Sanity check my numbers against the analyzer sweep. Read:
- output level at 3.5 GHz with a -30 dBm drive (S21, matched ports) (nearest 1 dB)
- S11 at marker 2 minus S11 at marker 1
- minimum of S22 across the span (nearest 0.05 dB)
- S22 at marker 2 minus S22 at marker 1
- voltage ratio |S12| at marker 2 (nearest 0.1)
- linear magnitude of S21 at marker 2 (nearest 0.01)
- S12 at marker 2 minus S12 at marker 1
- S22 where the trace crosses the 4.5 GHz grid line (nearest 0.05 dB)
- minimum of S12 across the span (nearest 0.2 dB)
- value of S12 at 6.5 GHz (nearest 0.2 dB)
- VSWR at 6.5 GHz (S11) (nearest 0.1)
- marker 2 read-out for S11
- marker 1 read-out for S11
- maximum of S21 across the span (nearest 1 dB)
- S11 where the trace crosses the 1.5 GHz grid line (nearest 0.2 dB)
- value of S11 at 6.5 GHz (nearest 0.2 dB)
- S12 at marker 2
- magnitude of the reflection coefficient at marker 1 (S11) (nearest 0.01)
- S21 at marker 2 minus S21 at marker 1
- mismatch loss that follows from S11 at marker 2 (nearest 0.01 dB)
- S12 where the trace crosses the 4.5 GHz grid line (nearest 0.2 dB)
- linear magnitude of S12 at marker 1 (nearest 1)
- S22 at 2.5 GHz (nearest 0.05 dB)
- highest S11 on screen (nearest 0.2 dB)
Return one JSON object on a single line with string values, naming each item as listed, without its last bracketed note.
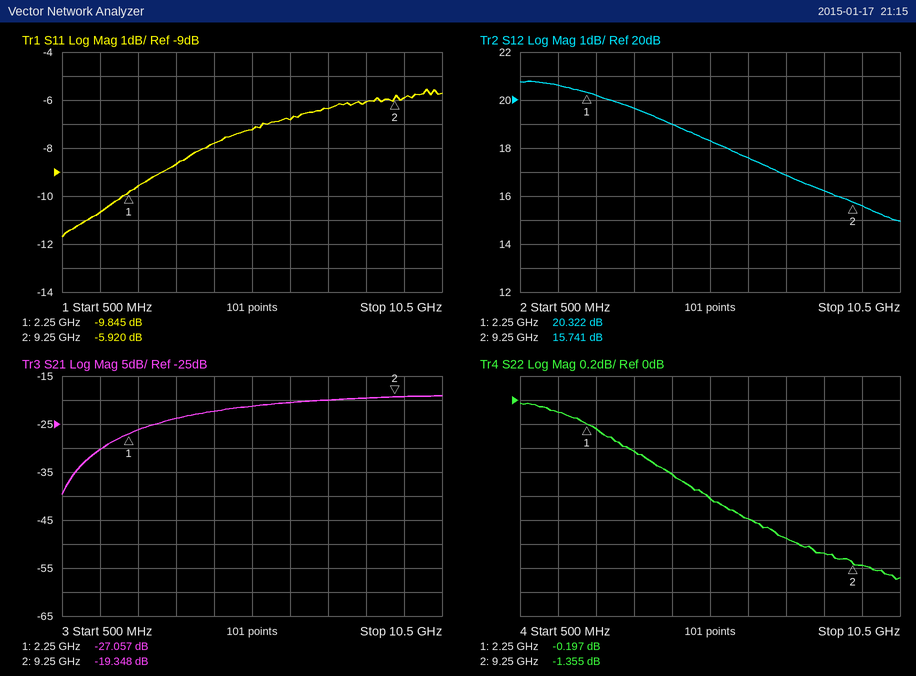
{"output level at 3.5 GHz with a -30 dBm drive (S21, matched ports)": "-54 dBm", "S11 at marker 2 minus S11 at marker 1": "3.925 dB", "minimum of S22 across the span": "-1.50 dB", "S22 at marker 2 minus S22 at marker 1": "-1.158 dB", "voltage ratio |S12| at marker 2": "6.1", "linear magnitude of S21 at marker 2": "0.11", "S12 at marker 2 minus S12 at marker 1": "-4.581 dB", "S22 where the trace crosses the 4.5 GHz grid line": "-0.60 dB", "minimum of S12 across the span": "15.0 dB", "value of S12 at 6.5 GHz": "17.6 dB", "VSWR at 6.5 GHz (S11)": "2.7", "marker 2 read-out for S11": "-5.920 dB", "marker 1 read-out for S11": "-9.845 dB", "maximum of S21 across the span": "-19 dB", "S11 where the trace crosses the 1.5 GHz grid line": "-10.6 dB", "value of S11 at 6.5 GHz": "-6.8 dB", "S12 at marker 2": "15.741 dB", "magnitude of the reflection coefficient at marker 1 (S11)": "0.32", "S21 at marker 2 minus S21 at marker 1": "7.709 dB", "mismatch loss that follows from S11 at marker 2": "1.28 dB", "S12 where the trace crosses the 4.5 GHz grid line": "19.0 dB", "linear magnitude of S12 at marker 1": "10", "S22 at 2.5 GHz": "-0.25 dB", "highest S11 on screen": "-5.6 dB"}
